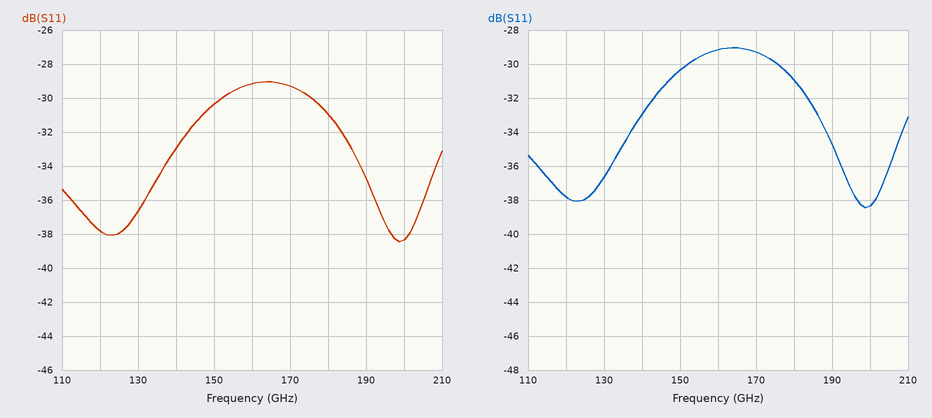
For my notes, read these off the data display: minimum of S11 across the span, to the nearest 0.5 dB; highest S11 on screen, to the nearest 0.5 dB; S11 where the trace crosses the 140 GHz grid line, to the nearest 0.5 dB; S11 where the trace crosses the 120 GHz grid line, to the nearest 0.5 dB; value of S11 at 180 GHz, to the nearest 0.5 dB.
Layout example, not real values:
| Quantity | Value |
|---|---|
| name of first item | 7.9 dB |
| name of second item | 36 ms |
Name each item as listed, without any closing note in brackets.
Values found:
| Quantity | Value |
|---|---|
| minimum of S11 across the span, to the nearest 0.5 dB | -38.5 dB |
| highest S11 on screen, to the nearest 0.5 dB | -29.0 dB |
| S11 where the trace crosses the 140 GHz grid line, to the nearest 0.5 dB | -33.0 dB |
| S11 where the trace crosses the 120 GHz grid line, to the nearest 0.5 dB | -38.0 dB |
| value of S11 at 180 GHz, to the nearest 0.5 dB | -31.0 dB |
